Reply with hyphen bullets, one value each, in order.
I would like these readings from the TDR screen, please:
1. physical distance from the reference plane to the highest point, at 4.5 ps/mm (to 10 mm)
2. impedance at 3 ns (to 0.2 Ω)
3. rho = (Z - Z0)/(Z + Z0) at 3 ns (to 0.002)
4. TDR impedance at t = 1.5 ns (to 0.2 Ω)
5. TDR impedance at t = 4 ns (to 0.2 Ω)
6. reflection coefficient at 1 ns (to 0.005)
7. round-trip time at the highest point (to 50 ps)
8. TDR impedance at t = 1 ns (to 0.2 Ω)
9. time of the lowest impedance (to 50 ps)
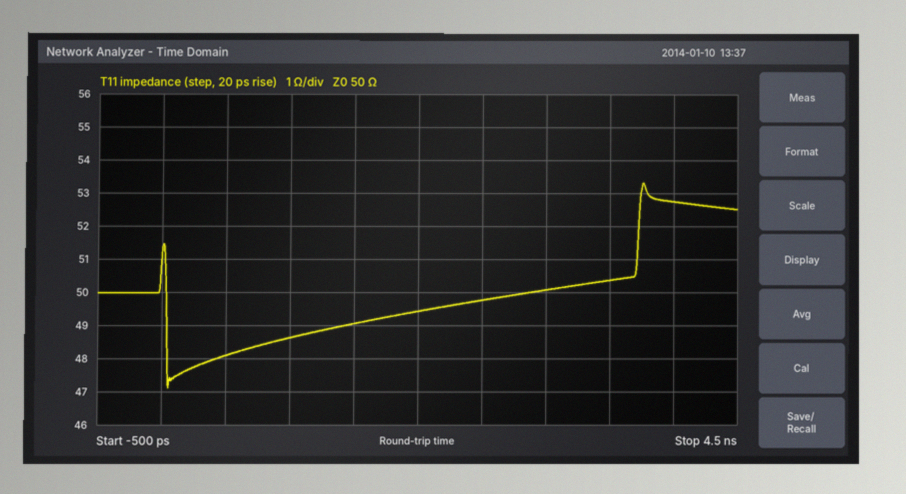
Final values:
- 420 mm
- 50.0 Ω
- 0.000
- 49.0 Ω
- 52.8 Ω
- -0.015
- 3.75 ns
- 48.6 Ω
- 50 ps
